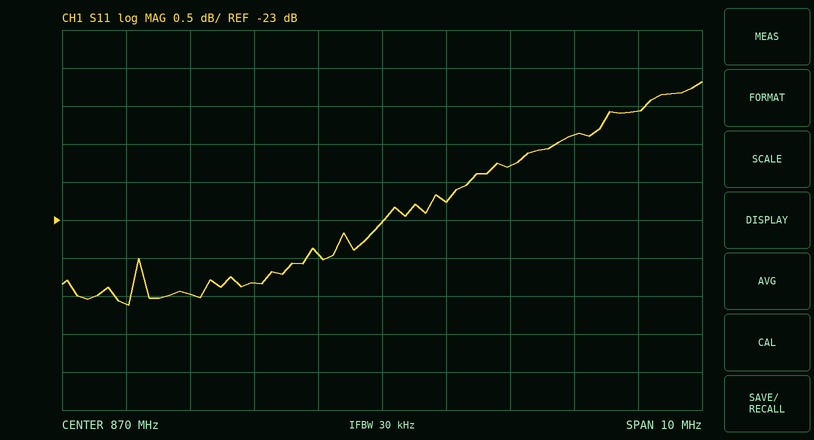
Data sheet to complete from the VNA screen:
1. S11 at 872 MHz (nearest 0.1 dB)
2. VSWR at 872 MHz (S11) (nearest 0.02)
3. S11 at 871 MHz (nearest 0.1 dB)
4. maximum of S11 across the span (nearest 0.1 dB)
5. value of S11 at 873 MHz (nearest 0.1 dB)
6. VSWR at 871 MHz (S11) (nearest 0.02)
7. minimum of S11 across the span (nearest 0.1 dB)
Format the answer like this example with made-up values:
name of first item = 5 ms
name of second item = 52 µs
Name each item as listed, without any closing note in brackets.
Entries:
S11 at 872 MHz = -22.3 dB
VSWR at 872 MHz (S11) = 1.16
S11 at 871 MHz = -22.8 dB
maximum of S11 across the span = -21.2 dB
value of S11 at 873 MHz = -21.9 dB
VSWR at 871 MHz (S11) = 1.16
minimum of S11 across the span = -24.1 dB
